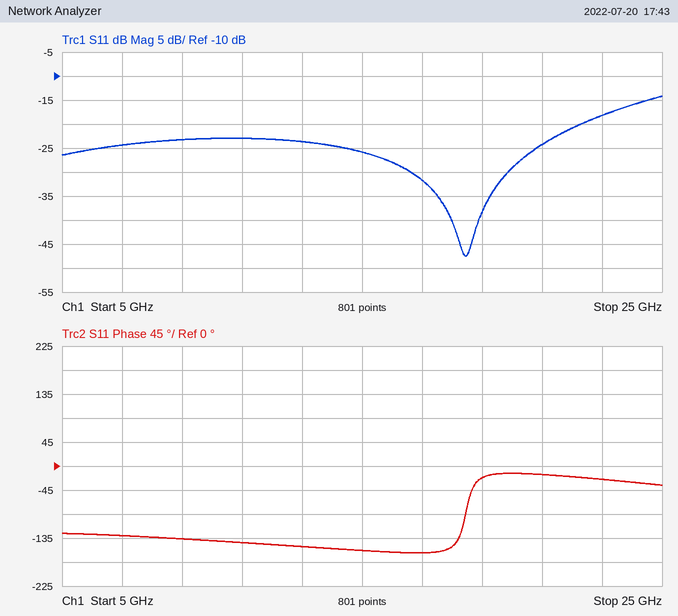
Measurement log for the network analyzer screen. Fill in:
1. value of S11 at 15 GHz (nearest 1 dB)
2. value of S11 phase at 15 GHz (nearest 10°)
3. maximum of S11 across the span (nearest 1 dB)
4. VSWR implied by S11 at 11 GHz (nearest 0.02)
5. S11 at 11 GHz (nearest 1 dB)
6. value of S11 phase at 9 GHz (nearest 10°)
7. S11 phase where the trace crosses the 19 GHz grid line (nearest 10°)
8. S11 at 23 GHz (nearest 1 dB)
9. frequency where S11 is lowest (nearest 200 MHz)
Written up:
-26 dB
-160°
-14 dB
1.16
-23 dB
-140°
-20°
-18 dB
18.4 GHz
